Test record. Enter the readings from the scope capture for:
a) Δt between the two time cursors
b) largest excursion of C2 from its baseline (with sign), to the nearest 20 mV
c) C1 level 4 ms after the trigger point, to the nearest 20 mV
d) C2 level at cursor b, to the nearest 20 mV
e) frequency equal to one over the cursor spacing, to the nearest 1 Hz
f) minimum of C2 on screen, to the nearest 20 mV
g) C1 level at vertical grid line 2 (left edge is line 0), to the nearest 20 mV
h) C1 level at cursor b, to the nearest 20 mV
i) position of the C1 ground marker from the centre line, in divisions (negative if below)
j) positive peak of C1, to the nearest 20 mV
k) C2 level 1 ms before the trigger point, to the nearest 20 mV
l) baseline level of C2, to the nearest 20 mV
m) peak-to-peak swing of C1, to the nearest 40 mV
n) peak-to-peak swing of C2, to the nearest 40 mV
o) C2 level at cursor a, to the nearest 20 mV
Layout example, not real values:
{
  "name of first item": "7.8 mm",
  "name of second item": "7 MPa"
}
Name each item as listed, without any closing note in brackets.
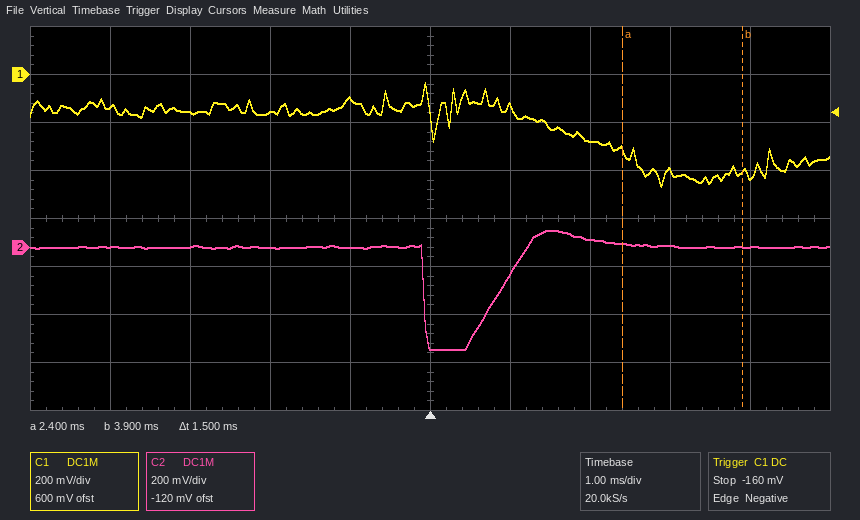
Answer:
{
  "Δt between the two time cursors": "1.5 ms",
  "largest excursion of C2 from its baseline (with sign), to the nearest 20 mV": "-420 mV",
  "C1 level 4 ms after the trigger point, to the nearest 20 mV": "-420 mV",
  "C2 level at cursor b, to the nearest 20 mV": "0 mV",
  "frequency equal to one over the cursor spacing, to the nearest 1 Hz": "667 Hz",
  "minimum of C2 on screen, to the nearest 20 mV": "-420 mV",
  "C1 level at vertical grid line 2 (left edge is line 0), to the nearest 20 mV": "-160 mV",
  "C1 level at cursor b, to the nearest 20 mV": "-400 mV",
  "position of the C1 ground marker from the centre line, in divisions": "+3.0 div",
  "positive peak of C1, to the nearest 20 mV": "-40 mV",
  "C2 level 1 ms before the trigger point, to the nearest 20 mV": "0 mV",
  "baseline level of C2, to the nearest 20 mV": "0 mV",
  "peak-to-peak swing of C1, to the nearest 40 mV": "440 mV",
  "peak-to-peak swing of C2, to the nearest 40 mV": "480 mV",
  "C2 level at cursor a, to the nearest 20 mV": "20 mV"
}
